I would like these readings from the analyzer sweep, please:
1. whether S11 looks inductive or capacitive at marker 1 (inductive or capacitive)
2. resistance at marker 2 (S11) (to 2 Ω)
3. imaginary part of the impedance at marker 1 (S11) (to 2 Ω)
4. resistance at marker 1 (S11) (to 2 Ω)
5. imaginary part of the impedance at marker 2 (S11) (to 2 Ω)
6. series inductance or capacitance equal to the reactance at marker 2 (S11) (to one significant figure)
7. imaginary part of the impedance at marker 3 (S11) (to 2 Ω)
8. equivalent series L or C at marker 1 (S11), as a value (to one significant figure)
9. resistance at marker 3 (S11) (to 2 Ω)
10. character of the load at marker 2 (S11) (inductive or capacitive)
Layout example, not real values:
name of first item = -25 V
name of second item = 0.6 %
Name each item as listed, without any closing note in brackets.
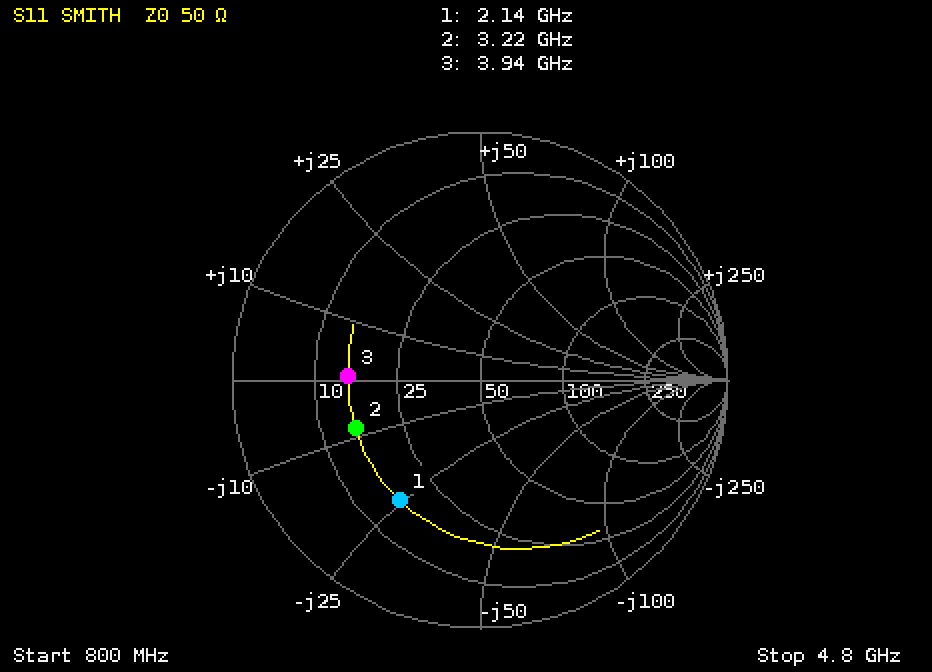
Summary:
whether S11 looks inductive or capacitive at marker 1 = capacitive
resistance at marker 2 (S11) = 16 Ω
imaginary part of the impedance at marker 1 (S11) = -24 Ω
resistance at marker 1 (S11) = 16 Ω
imaginary part of the impedance at marker 2 (S11) = -8 Ω
series inductance or capacitance equal to the reactance at marker 2 (S11) = 6 pF
imaginary part of the impedance at marker 3 (S11) = 0 Ω
equivalent series L or C at marker 1 (S11), as a value = 3 pF
resistance at marker 3 (S11) = 16 Ω
character of the load at marker 2 (S11) = capacitive
